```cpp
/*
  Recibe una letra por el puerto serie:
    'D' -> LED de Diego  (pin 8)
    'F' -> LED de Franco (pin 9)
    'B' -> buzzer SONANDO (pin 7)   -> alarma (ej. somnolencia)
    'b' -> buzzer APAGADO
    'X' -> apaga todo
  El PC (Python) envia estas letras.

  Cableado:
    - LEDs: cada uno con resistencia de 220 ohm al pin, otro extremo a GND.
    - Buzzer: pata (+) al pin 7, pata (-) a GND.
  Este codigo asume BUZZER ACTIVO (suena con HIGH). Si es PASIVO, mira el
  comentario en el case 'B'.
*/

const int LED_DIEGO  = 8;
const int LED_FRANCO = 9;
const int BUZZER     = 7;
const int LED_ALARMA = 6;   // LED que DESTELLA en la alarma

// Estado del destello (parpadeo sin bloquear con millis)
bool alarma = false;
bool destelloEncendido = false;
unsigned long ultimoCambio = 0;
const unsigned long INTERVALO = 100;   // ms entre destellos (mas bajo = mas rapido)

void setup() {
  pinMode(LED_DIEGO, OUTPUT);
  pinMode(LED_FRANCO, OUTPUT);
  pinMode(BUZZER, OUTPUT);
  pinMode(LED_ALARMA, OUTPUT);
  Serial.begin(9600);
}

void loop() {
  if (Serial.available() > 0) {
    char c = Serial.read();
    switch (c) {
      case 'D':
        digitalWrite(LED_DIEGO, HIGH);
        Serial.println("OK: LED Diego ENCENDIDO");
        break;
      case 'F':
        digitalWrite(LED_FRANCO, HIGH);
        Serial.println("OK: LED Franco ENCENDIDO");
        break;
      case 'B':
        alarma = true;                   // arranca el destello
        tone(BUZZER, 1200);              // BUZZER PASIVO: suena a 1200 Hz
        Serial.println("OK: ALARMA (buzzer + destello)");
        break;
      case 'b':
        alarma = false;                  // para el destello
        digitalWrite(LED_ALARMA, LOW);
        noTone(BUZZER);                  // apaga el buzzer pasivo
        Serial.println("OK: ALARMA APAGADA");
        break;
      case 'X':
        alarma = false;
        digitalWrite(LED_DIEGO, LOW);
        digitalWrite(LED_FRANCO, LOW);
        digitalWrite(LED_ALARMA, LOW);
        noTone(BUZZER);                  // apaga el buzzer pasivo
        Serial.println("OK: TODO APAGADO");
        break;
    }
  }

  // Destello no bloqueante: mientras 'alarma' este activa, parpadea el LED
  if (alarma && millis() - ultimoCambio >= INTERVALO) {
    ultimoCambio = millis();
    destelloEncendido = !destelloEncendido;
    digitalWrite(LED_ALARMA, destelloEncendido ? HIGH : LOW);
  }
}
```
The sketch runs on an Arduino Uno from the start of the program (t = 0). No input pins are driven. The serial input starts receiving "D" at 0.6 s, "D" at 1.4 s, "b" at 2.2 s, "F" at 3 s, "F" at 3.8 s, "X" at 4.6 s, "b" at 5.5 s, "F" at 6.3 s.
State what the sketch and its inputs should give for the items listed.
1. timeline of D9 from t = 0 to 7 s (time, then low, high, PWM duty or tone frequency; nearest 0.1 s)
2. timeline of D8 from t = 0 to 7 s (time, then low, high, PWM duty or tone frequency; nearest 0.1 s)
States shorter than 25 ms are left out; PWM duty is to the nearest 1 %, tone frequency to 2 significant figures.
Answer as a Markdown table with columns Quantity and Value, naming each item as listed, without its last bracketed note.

| Quantity | Value |
|---|---|
| timeline of D9 from t = 0 to 7 s | 0 s low; 3 s high; 4.6 s low; 6.3 s high |
| timeline of D8 from t = 0 to 7 s | 0 s low; 0.6 s high; 4.6 s low |
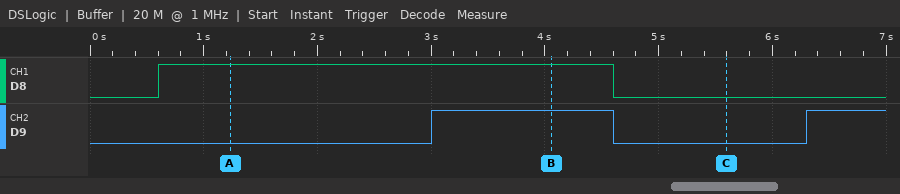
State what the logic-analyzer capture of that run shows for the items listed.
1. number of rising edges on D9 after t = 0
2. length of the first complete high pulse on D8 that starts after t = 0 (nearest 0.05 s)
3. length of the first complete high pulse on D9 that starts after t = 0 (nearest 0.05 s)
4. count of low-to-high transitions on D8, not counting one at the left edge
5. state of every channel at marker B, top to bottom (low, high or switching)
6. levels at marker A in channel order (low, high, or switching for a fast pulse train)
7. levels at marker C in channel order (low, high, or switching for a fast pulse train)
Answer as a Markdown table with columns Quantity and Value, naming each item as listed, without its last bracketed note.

| Quantity | Value |
|---|---|
| number of rising edges on D9 after t = 0 | 2 |
| length of the first complete high pulse on D8 that starts after t = 0 | 4.00 s |
| length of the first complete high pulse on D9 that starts after t = 0 | 1.60 s |
| count of low-to-high transitions on D8, not counting one at the left edge | 1 |
| state of every channel at marker B, top to bottom | D8 high, D9 high |
| levels at marker A in channel order | D8 high, D9 low |
| levels at marker C in channel order | D8 low, D9 low |
